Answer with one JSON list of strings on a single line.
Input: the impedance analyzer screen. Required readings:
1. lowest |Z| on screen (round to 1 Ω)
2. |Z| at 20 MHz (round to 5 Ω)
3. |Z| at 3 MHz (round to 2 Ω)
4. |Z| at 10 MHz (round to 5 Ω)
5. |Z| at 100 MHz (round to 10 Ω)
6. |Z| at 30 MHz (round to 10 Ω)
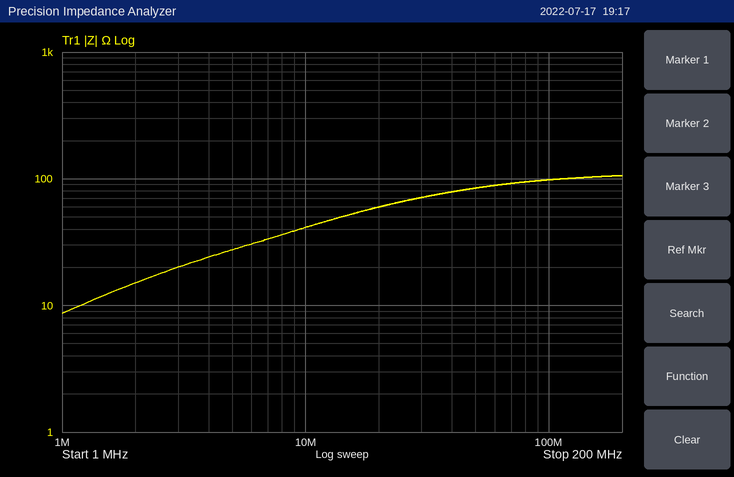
["9 Ω", "60 Ω", "20 Ω", "40 Ω", "100 Ω", "70 Ω"]
